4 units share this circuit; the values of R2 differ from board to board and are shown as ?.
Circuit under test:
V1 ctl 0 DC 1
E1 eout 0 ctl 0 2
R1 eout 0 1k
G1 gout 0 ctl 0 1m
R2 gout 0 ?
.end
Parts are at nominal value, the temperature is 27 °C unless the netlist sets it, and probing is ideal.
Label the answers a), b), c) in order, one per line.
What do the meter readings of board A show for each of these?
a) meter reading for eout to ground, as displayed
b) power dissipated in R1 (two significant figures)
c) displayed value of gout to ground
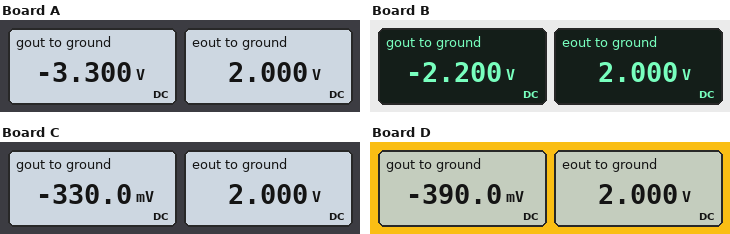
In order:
a) 2.000 V
b) 4.0 mW
c) -3.300 V
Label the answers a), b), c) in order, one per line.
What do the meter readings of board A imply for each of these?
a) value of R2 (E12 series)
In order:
a) 3.3 kΩ
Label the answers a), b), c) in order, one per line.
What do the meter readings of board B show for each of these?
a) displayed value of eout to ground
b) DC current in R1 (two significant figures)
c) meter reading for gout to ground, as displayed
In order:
a) 2.000 V
b) 2.0 mA
c) -2.200 V
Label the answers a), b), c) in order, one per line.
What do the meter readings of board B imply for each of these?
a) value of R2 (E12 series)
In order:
a) 2.2 kΩ
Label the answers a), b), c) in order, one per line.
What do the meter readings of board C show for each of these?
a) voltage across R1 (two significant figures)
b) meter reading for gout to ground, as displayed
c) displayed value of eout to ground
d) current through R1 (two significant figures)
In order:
a) 2.0 V
b) -330.0 mV
c) 2.000 V
d) 2.0 mA
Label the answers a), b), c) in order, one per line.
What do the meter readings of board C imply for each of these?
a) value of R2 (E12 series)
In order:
a) 330 Ω
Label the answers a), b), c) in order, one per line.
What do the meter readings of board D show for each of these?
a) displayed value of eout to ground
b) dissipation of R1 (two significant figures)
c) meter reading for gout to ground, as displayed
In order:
a) 2.000 V
b) 4.0 mW
c) -390.0 mV
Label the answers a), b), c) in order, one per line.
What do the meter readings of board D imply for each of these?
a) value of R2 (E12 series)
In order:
a) 390 Ω
